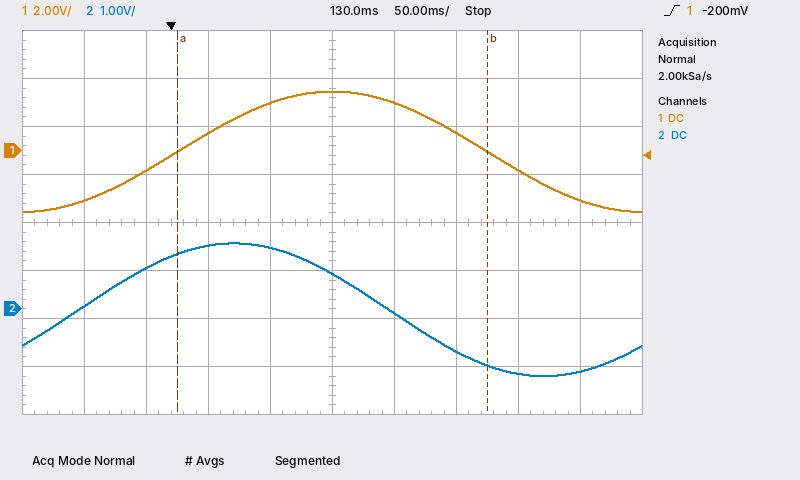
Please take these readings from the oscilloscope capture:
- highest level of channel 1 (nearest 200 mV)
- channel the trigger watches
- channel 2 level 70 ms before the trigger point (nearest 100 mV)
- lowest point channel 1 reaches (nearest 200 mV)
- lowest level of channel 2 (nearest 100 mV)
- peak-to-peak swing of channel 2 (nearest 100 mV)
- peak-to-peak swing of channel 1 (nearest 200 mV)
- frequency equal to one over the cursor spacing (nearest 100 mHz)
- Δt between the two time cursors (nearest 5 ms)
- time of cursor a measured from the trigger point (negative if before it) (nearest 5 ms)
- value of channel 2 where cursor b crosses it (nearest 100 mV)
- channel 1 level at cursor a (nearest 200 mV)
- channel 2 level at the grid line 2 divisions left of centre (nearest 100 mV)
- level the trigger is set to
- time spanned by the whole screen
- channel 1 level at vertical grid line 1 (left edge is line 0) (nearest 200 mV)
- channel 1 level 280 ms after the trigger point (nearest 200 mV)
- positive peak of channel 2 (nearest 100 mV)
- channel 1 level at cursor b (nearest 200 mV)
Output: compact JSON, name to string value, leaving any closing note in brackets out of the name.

{"highest level of channel 1": "2.4 V", "channel the trigger watches": "channel 1", "channel 2 level 70 ms before the trigger point": "100 mV", "lowest point channel 1 reaches": "-2.6 V", "lowest level of channel 2": "-1.4 V", "peak-to-peak swing of channel 2": "2.8 V", "peak-to-peak swing of channel 1": "5.0 V", "frequency equal to one over the cursor spacing": "4.0 Hz", "Δt between the two time cursors": "250 ms", "time of cursor a measured from the trigger point (negative if before it)": "+5 ms", "value of channel 2 where cursor b crosses it": "-1.2 V", "channel 1 level at cursor a": "0.0 V", "channel 2 level at the grid line 2 divisions left of centre": "1.3 V", "level the trigger is set to": "-200 mV", "time spanned by the whole screen": "500 ms", "channel 1 level at vertical grid line 1 (left edge is line 0)": "-2.0 V", "channel 1 level 280 ms after the trigger point": "-800 mV", "positive peak of channel 2": "1.4 V", "channel 1 level at cursor b": "0.0 V"}
